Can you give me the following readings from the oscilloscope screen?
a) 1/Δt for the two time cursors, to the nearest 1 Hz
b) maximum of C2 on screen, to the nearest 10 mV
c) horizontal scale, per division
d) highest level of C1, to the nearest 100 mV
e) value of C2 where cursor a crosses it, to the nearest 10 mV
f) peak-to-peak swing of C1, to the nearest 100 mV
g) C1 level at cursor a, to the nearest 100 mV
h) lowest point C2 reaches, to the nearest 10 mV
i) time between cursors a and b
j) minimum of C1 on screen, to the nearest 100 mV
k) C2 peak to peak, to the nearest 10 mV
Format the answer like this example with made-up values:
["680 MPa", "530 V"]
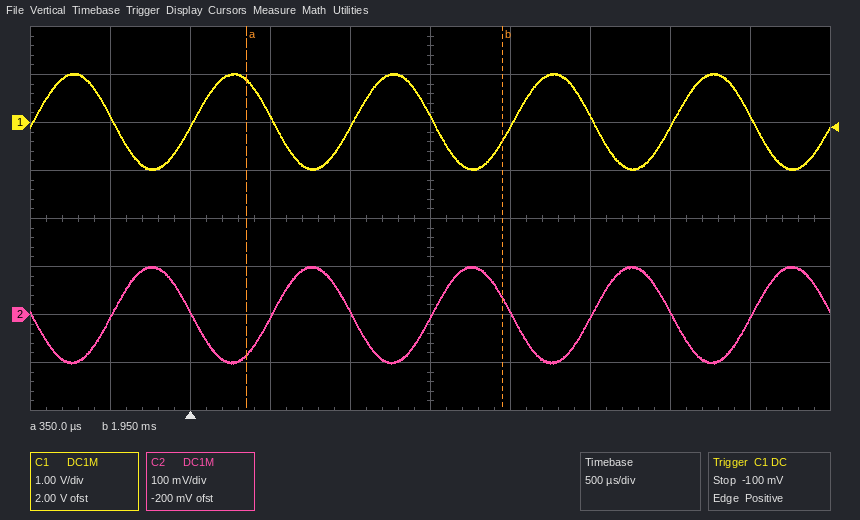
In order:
["625 Hz", "100 mV", "500 µs", "1.0 V", "-80 mV", "2.0 V", "900 mV", "-100 mV", "1.60 ms", "-1.0 V", "200 mV"]
